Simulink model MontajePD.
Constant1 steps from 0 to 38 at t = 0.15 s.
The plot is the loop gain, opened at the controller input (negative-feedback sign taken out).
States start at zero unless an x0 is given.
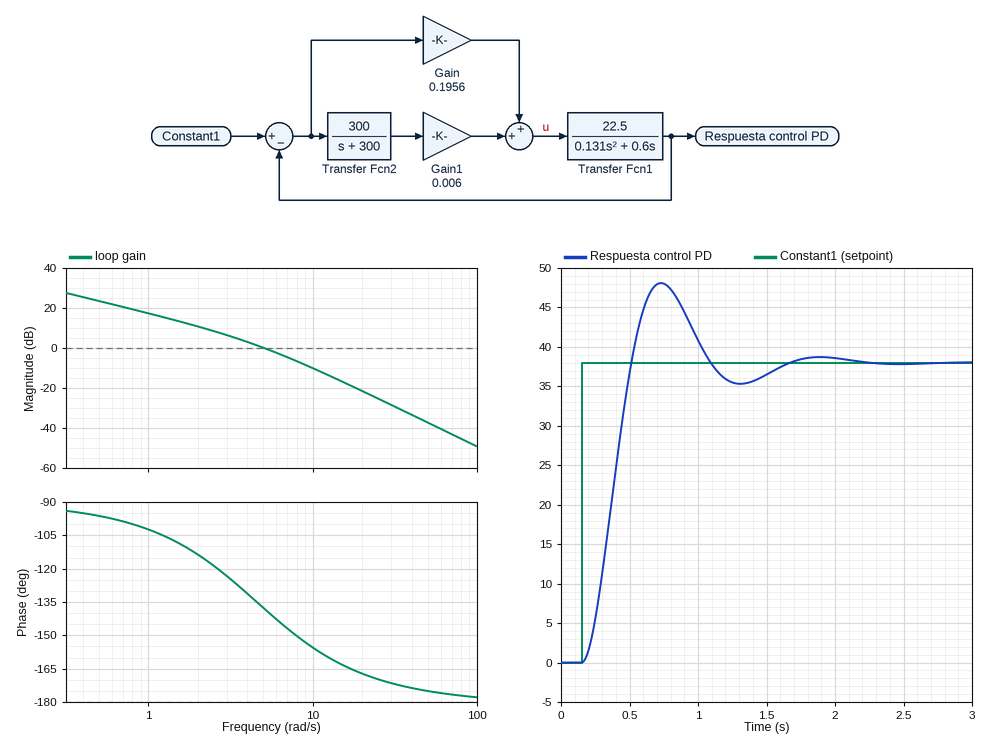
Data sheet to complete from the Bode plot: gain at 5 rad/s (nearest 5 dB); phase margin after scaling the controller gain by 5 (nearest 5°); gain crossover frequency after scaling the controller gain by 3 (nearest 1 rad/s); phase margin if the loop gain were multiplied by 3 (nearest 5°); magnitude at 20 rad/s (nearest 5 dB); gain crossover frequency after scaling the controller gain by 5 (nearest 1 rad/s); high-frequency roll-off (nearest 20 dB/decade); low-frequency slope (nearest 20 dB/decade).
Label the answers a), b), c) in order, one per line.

a) 0 dB
b) 20°
c) 10 rad/s
d) 25°
e) -20 dB
f) 13 rad/s
g) -40 dB/decade
h) -20 dB/decade
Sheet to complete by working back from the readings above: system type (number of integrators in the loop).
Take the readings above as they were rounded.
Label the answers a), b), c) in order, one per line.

a) 1
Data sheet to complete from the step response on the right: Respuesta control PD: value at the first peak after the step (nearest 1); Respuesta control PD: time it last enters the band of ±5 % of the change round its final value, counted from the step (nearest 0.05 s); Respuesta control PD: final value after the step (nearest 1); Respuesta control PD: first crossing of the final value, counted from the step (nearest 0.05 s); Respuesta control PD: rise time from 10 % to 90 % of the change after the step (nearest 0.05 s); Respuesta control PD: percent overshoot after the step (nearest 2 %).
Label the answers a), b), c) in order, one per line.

a) 48
b) 1.30 s
c) 38
d) 0.35 s
e) 0.25 s
f) 26 %
